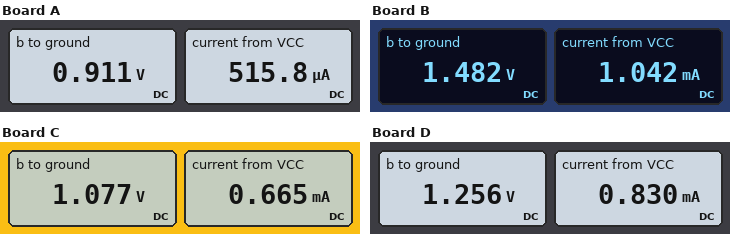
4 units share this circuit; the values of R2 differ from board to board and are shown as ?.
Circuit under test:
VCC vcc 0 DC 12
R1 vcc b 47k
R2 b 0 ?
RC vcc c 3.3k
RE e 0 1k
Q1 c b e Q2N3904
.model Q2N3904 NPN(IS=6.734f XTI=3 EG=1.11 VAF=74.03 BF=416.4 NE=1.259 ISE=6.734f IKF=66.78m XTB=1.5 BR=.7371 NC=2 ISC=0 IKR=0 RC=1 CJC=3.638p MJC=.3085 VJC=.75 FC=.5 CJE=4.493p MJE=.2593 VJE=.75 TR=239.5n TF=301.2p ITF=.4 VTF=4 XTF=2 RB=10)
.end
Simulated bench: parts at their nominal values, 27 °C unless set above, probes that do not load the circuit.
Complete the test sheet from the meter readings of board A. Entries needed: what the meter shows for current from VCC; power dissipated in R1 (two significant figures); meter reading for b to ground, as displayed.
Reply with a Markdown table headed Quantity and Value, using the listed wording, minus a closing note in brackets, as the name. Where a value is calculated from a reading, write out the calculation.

| Quantity | Value |
|---|---|
| what the meter shows for current from VCC | 515.8 µA |
| power dissipated in R1 | (12 V - 911 mV)^2 / 47 kΩ = 2.6 mW |
| meter reading for b to ground, as displayed | 0.911 V |
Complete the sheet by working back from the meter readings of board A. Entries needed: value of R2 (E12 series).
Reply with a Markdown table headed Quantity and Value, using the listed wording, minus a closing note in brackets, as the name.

| Quantity | Value |
|---|---|
| value of R2 | 3.9 kΩ |
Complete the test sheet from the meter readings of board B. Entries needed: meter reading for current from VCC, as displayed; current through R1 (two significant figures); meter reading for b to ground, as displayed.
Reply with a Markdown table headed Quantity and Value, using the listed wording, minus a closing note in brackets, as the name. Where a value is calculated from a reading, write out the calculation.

| Quantity | Value |
|---|---|
| meter reading for current from VCC, as displayed | 1.042 mA |
| current through R1 | (12 V - 1.482 V) / 47 kΩ = 220 µA |
| meter reading for b to ground, as displayed | 1.482 V |
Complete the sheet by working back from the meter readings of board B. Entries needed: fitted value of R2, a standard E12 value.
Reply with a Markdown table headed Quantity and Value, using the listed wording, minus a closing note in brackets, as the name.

| Quantity | Value |
|---|---|
| fitted value of R2, a standard E12 value | 6.8 kΩ |
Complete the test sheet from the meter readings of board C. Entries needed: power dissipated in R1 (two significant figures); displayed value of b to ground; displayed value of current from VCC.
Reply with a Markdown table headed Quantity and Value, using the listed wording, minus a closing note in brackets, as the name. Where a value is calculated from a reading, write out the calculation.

| Quantity | Value |
|---|---|
| power dissipated in R1 | (12 V - 1.077 V)^2 / 47 kΩ = 2.5 mW |
| displayed value of b to ground | 1.077 V |
| displayed value of current from VCC | 0.665 mA |
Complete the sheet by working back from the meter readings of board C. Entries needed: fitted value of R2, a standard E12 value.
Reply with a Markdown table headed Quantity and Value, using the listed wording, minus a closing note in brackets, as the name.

| Quantity | Value |
|---|---|
| fitted value of R2, a standard E12 value | 4.7 kΩ |
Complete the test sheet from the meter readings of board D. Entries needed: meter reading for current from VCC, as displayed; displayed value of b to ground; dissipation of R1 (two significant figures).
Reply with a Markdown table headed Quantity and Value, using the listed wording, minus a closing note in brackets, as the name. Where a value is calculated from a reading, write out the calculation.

| Quantity | Value |
|---|---|
| meter reading for current from VCC, as displayed | 0.830 mA |
| displayed value of b to ground | 1.256 V |
| dissipation of R1 | (12 V - 1.256 V)^2 / 47 kΩ = 2.5 mW |
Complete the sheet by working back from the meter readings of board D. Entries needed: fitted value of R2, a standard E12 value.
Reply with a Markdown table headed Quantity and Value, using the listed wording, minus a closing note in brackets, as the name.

| Quantity | Value |
|---|---|
| fitted value of R2, a standard E12 value | 5.6 kΩ |
